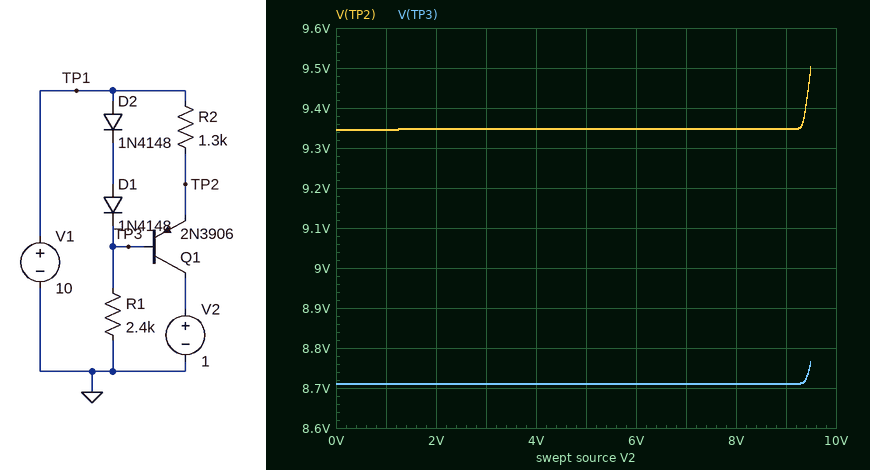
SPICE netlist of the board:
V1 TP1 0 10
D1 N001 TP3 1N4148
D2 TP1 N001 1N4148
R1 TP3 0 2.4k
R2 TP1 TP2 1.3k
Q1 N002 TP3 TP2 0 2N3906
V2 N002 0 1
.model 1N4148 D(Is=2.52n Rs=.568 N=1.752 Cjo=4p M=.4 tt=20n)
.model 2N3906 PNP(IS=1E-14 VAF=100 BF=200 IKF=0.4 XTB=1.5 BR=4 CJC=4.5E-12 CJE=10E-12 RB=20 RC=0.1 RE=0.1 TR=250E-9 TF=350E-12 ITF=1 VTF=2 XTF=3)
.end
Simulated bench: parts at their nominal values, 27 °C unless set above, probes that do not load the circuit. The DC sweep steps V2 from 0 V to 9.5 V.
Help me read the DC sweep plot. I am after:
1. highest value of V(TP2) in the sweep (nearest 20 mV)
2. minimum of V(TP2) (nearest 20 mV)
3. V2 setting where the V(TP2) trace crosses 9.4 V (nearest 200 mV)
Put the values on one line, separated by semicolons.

9.50 V; 9.34 V; 9.4 V
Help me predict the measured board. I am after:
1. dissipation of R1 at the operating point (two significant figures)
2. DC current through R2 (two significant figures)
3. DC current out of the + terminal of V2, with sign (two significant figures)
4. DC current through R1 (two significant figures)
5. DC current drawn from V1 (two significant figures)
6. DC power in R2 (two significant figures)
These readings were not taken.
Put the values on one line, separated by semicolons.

32 mW; 500 µA; -500 µA; 3.6 mA; 4.1 mA; 330 µW
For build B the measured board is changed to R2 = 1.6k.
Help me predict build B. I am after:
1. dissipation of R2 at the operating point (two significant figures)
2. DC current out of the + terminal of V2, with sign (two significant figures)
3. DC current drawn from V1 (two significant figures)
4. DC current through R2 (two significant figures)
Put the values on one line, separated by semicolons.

270 µW; -410 µA; 4.0 mA; 410 µA
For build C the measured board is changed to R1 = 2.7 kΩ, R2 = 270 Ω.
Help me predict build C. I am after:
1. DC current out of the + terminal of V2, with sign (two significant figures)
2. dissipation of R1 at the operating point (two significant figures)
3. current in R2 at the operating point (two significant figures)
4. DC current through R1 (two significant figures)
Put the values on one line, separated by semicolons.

-2.2 mA; 28 mW; 2.2 mA; 3.2 mA
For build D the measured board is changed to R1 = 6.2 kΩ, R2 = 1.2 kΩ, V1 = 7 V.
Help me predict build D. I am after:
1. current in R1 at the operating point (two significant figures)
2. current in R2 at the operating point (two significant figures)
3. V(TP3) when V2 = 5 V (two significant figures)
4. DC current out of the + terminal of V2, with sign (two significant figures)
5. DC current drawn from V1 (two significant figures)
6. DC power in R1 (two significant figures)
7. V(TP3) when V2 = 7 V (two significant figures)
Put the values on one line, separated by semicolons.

940 µA; 440 µA; 5.8 V; -440 µA; 1.4 mA; 5.5 mW; 6.3 V
